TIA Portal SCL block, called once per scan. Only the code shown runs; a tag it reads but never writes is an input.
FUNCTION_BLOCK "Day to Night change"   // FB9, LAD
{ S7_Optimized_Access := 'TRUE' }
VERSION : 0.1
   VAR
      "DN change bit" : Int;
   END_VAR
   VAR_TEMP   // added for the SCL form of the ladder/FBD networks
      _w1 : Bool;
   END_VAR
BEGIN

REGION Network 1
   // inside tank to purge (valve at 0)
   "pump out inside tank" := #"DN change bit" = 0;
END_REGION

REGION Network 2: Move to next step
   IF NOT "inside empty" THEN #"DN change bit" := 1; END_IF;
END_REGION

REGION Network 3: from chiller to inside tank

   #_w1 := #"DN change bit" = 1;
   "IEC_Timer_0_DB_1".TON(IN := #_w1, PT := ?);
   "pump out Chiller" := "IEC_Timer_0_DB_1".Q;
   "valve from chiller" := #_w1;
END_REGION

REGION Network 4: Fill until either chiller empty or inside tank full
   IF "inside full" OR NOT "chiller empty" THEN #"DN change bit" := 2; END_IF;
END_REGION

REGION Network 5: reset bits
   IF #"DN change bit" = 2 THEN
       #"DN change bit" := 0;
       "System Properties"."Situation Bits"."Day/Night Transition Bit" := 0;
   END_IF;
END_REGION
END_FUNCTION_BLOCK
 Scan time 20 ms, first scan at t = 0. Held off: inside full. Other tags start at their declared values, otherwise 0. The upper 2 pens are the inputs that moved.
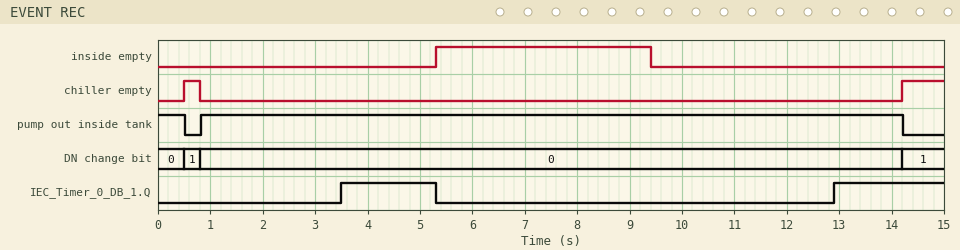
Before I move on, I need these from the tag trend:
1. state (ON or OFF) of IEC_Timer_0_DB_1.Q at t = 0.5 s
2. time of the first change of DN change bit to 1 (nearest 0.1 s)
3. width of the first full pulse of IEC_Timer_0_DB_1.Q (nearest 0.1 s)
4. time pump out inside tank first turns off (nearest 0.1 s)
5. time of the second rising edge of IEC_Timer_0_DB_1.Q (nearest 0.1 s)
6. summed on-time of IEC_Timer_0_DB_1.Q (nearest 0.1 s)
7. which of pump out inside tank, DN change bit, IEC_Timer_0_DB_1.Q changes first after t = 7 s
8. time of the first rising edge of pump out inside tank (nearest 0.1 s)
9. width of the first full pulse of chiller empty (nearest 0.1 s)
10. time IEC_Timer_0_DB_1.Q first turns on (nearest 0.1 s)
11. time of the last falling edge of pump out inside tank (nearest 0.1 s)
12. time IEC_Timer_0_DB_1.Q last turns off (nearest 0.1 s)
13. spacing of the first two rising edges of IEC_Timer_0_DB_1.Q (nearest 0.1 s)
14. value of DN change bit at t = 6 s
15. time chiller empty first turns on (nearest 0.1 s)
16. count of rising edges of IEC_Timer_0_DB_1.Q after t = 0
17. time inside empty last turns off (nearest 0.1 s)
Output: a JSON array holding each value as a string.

["OFF", "0.5 s", "1.8 s", "0.5 s", "12.9 s", "3.9 s", "IEC_Timer_0_DB_1.Q", "0.8 s", "0.3 s", "3.5 s", "14.2 s", "5.3 s", "9.4 s", "0", "0.5 s", "2", "9.4 s"]
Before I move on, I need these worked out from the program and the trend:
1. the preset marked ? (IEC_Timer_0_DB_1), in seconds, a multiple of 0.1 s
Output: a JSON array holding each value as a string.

["3.5 s"]
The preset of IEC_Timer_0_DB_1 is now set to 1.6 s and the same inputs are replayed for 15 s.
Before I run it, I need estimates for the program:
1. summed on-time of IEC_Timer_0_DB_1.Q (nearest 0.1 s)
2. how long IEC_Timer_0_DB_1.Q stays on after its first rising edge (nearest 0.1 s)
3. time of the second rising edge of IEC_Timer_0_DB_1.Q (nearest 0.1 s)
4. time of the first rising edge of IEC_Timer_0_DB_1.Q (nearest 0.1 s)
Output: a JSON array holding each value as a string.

["7.7 s", "3.7 s", "11.0 s", "1.6 s"]
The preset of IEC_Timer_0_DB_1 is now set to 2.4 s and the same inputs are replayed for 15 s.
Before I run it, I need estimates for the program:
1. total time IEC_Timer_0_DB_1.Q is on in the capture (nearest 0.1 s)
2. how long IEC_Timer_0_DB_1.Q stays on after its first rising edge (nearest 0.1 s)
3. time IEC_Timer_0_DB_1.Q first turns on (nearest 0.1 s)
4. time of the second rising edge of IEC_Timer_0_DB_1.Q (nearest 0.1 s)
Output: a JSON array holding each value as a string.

["6.1 s", "2.9 s", "2.4 s", "11.8 s"]
